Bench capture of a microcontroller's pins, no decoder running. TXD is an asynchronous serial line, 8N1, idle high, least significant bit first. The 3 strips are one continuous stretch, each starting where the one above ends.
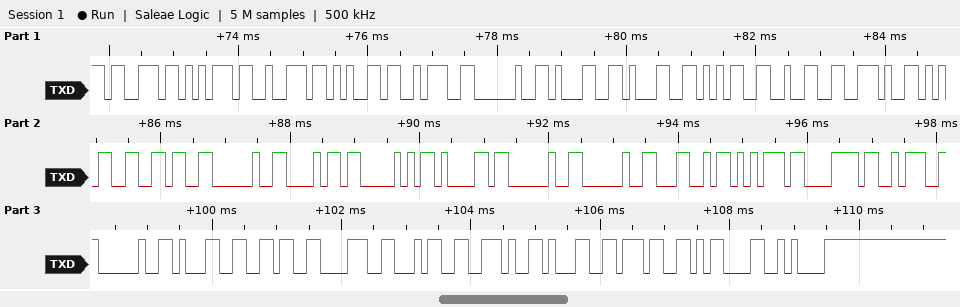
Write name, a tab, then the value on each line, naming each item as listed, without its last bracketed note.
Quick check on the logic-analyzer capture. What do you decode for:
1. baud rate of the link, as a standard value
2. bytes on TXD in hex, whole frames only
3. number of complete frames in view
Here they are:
baud rate of the link, as a standard value	9600 baud
bytes on TXD in hex, whole frames only	73 75 72 65 3A 20 31 31 35 32 2E 35 36 20 68 50 61 20 20 4C 75 78 3A 20 31 36 38 34 2E 31 37 0D 0A
number of complete frames in view	33
